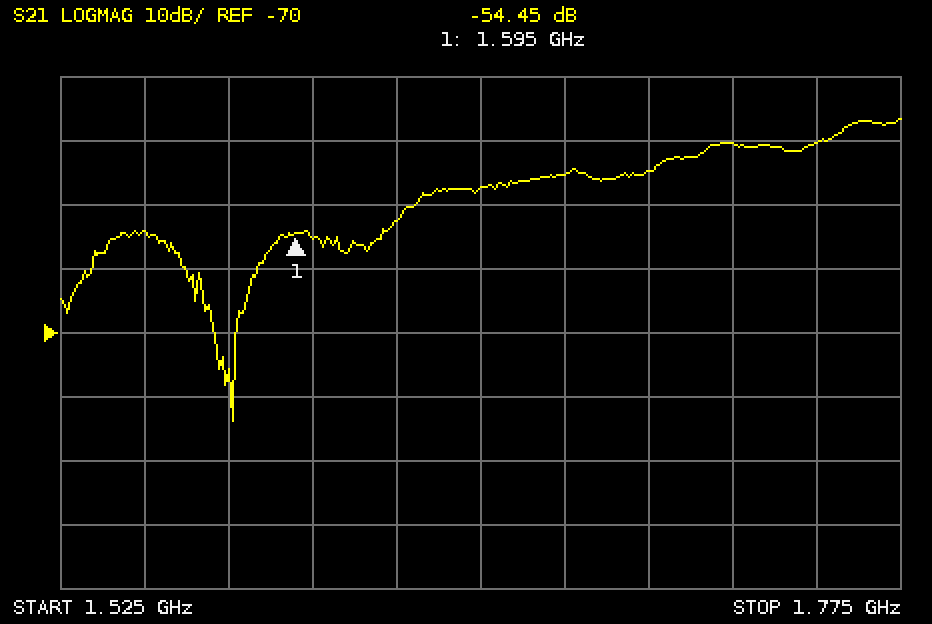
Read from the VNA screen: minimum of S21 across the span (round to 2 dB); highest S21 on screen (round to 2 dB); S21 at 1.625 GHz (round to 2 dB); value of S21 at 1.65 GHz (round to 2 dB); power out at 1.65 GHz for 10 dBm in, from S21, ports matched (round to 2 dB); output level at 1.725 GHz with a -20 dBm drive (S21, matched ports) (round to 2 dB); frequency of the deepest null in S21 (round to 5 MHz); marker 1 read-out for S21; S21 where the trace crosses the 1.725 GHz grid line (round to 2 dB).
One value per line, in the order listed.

-84 dB
-36 dB
-52 dB
-48 dB
-38 dBm
-60 dBm
1.575 GHz
-54.45 dB
-40 dB
